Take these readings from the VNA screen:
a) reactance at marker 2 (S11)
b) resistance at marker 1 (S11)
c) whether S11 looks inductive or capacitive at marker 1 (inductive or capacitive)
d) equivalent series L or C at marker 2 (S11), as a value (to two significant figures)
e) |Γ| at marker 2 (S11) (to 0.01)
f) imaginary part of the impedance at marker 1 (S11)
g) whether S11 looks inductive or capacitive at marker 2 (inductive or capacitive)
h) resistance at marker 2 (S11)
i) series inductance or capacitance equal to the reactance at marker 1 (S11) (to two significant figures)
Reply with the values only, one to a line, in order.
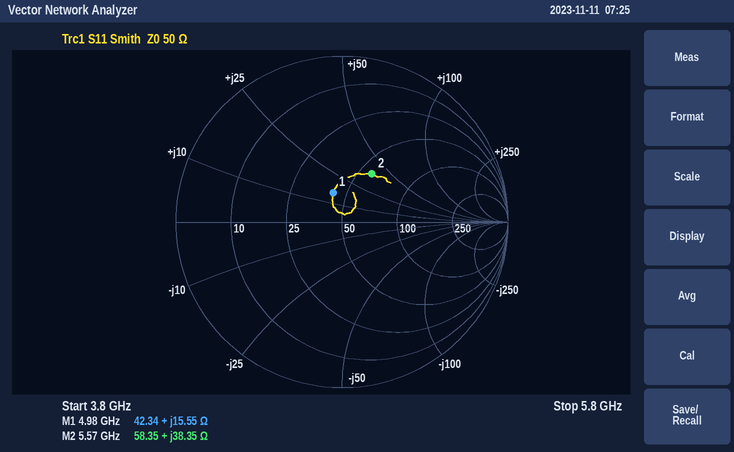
+38.35 Ω
42.34 Ω
inductive
1.1 nH
0.34
+15.55 Ω
inductive
58.35 Ω
500 pH
